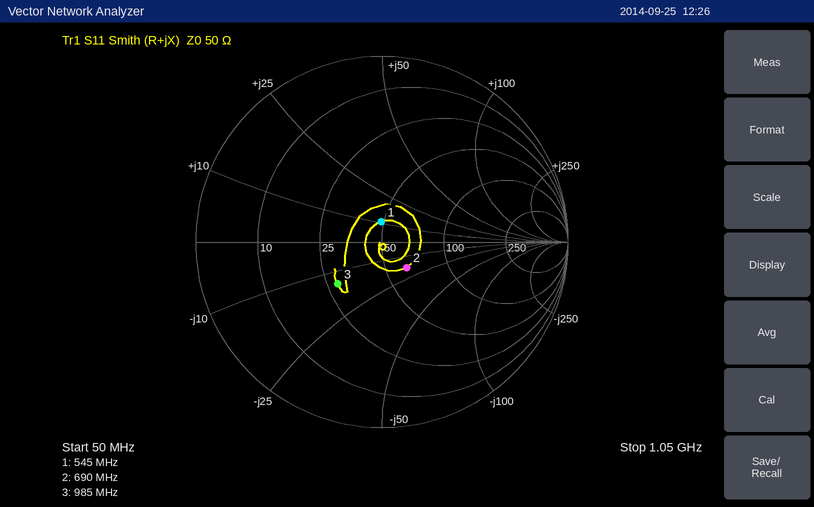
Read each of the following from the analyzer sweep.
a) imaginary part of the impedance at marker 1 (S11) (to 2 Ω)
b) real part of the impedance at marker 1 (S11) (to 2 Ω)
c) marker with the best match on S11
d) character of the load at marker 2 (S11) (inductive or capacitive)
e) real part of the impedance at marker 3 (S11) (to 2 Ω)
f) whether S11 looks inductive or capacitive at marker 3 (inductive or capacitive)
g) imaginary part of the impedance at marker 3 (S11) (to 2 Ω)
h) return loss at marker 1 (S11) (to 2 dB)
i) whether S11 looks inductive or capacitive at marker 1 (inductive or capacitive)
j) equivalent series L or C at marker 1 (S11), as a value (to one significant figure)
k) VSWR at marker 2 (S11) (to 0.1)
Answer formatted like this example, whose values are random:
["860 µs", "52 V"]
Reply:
["+10 Ω", "48 Ω", "marker 1", "capacitive", "28 Ω", "capacitive", "-14 Ω", "20 dB", "inductive", "3 nH", "1.5"]
